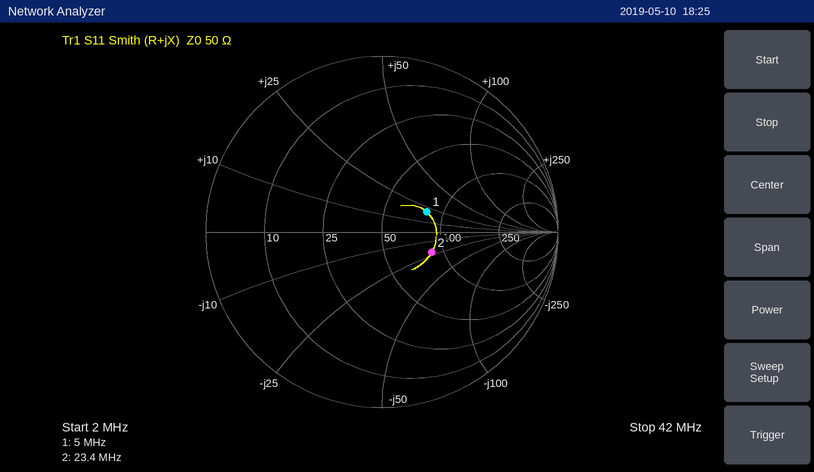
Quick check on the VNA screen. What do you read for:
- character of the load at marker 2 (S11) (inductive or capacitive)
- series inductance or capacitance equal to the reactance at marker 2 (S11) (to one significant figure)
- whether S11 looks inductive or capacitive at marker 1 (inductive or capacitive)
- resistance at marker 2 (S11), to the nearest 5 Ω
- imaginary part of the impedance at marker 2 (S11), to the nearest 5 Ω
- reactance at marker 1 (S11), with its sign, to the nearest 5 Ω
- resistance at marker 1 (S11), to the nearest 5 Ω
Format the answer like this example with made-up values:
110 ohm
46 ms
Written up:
capacitive
300 pF
inductive
85 Ω
-20 Ω
+20 Ω
80 Ω
